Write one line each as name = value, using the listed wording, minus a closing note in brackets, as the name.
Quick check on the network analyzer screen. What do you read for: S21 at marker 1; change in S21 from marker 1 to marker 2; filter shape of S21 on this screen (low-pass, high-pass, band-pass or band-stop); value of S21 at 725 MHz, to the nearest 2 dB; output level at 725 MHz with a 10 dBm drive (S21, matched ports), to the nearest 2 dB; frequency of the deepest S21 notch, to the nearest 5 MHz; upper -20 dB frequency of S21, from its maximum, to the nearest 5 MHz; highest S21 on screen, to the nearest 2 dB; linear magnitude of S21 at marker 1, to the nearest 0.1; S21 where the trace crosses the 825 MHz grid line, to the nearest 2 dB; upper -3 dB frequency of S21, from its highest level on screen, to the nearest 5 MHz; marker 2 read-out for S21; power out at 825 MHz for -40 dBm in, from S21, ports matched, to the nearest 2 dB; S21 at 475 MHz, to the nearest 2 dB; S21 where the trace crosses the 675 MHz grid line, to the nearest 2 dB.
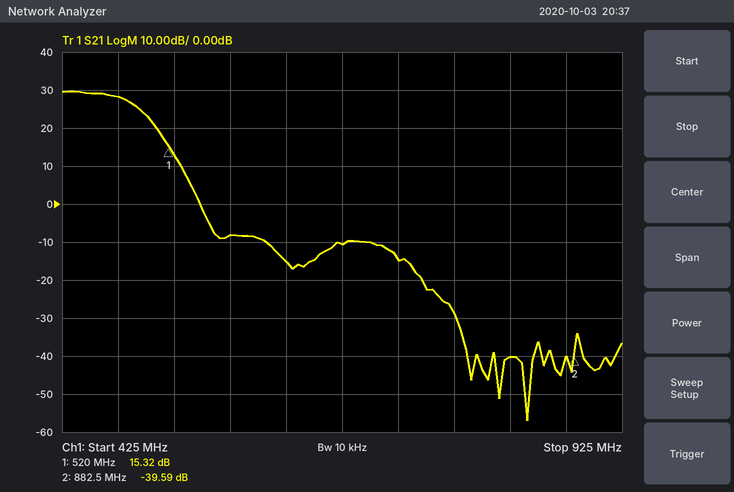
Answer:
S21 at marker 1 = 15.32 dB
change in S21 from marker 1 to marker 2 = -54.91 dB
filter shape of S21 on this screen = low-pass
value of S21 at 725 MHz, to the nearest 2 dB = -14 dB
output level at 725 MHz with a 10 dBm drive (S21, matched ports), to the nearest 2 dB = -4 dBm
frequency of the deepest S21 notch, to the nearest 5 MHz = 840 MHz
upper -20 dB frequency of S21, from its maximum, to the nearest 5 MHz = 530 MHz
highest S21 on screen, to the nearest 2 dB = 30 dB
linear magnitude of S21 at marker 1, to the nearest 0.1 = 5.8
S21 where the trace crosses the 825 MHz grid line, to the nearest 2 dB = -40 dB
upper -3 dB frequency of S21, from its highest level on screen, to the nearest 5 MHz = 485 MHz
marker 2 read-out for S21 = -39.59 dB
power out at 825 MHz for -40 dBm in, from S21, ports matched, to the nearest 2 dB = -80 dBm
S21 at 475 MHz, to the nearest 2 dB = 28 dB
S21 where the trace crosses the 675 MHz grid line, to the nearest 2 dB = -10 dB
